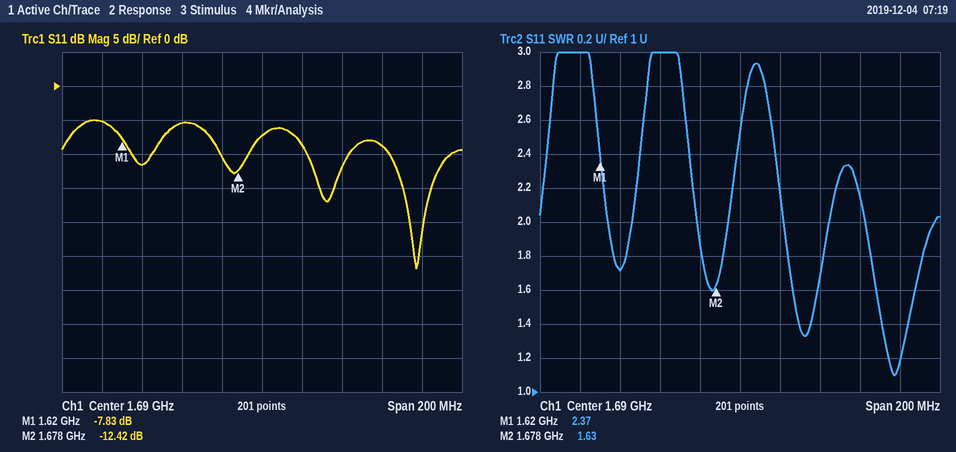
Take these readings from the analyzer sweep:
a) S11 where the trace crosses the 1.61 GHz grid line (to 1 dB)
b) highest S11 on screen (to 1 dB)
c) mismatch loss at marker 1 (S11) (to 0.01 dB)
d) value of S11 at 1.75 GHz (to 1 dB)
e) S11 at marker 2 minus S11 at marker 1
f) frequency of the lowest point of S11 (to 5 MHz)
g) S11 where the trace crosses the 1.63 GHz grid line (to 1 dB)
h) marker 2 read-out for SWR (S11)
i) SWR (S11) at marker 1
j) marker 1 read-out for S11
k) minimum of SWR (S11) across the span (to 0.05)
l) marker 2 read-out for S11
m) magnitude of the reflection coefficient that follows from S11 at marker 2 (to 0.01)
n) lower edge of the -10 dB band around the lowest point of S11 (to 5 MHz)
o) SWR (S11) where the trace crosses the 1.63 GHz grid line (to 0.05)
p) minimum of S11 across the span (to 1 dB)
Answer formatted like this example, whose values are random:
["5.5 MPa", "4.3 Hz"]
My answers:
["-5 dB", "-5 dB", "0.78 dB", "-9 dB", "-4.59 dB", "1.765 GHz", "-12 dB", "1.63", "2.37", "-7.83 dB", "1.10", "-12.42 dB", "0.24", "1.755 GHz", "1.70", "-27 dB"]
